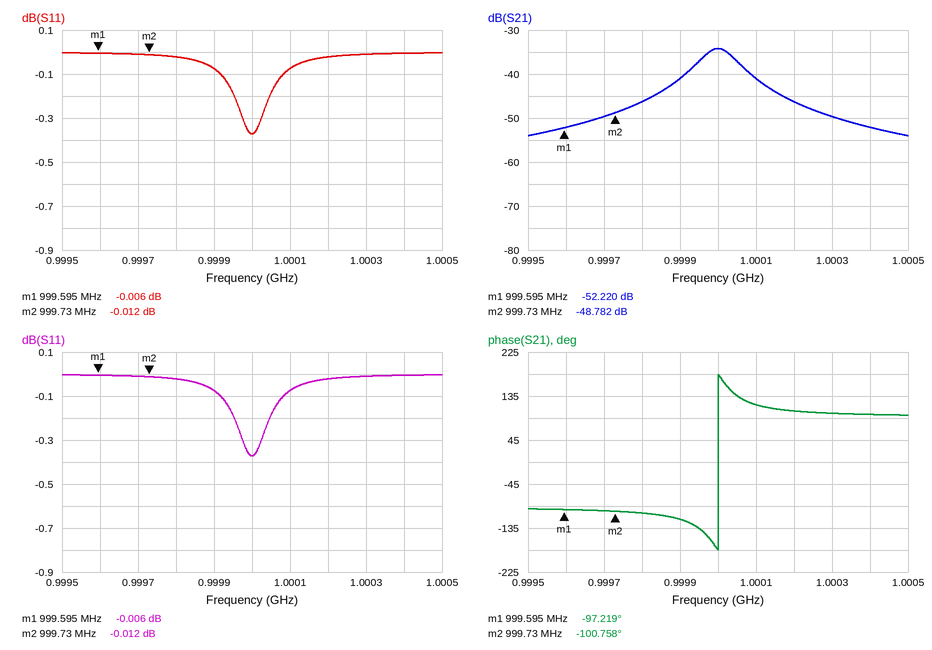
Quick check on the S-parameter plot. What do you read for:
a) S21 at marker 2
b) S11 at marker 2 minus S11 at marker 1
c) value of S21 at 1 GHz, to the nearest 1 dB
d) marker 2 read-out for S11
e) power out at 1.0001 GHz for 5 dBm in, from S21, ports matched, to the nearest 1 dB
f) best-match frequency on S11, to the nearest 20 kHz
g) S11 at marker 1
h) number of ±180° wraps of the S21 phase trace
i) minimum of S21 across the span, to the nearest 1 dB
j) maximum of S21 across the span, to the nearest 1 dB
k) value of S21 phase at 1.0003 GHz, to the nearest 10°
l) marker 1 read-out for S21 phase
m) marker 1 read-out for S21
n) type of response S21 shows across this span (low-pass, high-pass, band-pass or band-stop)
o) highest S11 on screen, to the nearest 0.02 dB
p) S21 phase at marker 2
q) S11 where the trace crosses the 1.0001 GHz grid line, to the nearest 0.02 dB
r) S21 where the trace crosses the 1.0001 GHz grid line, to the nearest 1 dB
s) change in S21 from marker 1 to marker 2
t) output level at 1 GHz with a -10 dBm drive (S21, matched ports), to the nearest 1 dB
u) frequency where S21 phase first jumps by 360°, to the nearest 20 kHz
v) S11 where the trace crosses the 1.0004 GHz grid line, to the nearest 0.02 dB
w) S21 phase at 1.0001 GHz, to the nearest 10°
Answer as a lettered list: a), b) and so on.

a) -48.782 dB
b) -0.006 dB
c) -34 dB
d) -0.012 dB
e) -36 dBm
f) 1.00000 GHz
g) -0.006 dB
h) 1
i) -54 dB
j) -34 dB
k) 100°
l) -97.219°
m) -52.220 dB
n) band-pass
o) 0.00 dB
p) -100.758°
q) -0.08 dB
r) -41 dB
s) 3.438 dB
t) -44 dBm
u) 1.00000 GHz
v) 0.00 dB
w) 120°
